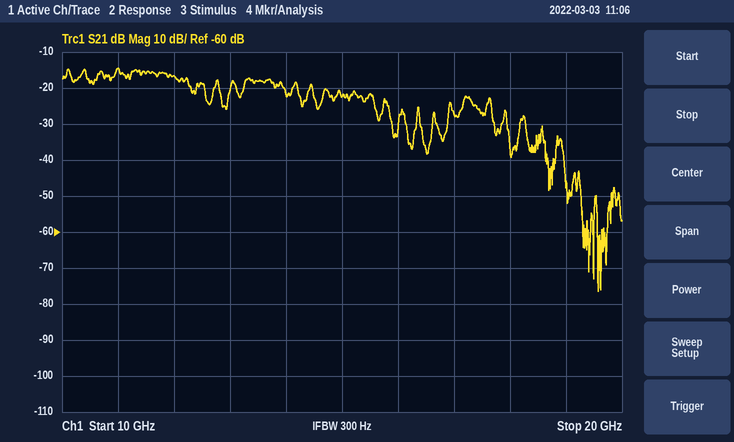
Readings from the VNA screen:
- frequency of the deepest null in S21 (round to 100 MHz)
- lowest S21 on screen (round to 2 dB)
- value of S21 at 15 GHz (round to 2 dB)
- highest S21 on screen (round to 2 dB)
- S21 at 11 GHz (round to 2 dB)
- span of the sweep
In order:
19.6 GHz
-76 dB
-22 dB
-14 dB
-14 dB
10 GHz
